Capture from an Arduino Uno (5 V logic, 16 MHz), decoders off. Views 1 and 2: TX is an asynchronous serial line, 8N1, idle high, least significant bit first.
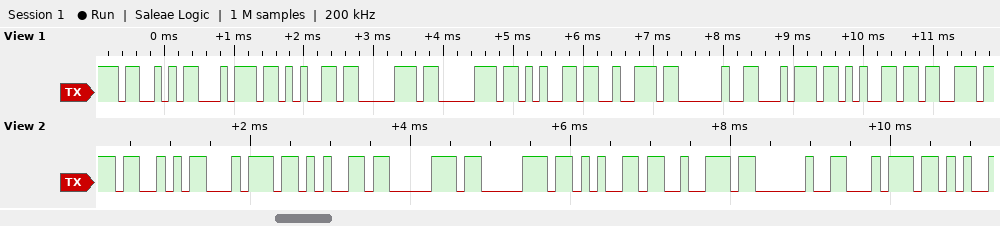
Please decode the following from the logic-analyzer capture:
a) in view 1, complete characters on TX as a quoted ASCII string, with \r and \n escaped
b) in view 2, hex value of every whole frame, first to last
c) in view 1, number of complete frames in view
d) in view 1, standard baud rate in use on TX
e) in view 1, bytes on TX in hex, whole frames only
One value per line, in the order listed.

"Stepper tes"
53 74 65 70 70 65 72 20 74
11
9600 baud
53 74 65 70 70 65 72 20 74 65 73
